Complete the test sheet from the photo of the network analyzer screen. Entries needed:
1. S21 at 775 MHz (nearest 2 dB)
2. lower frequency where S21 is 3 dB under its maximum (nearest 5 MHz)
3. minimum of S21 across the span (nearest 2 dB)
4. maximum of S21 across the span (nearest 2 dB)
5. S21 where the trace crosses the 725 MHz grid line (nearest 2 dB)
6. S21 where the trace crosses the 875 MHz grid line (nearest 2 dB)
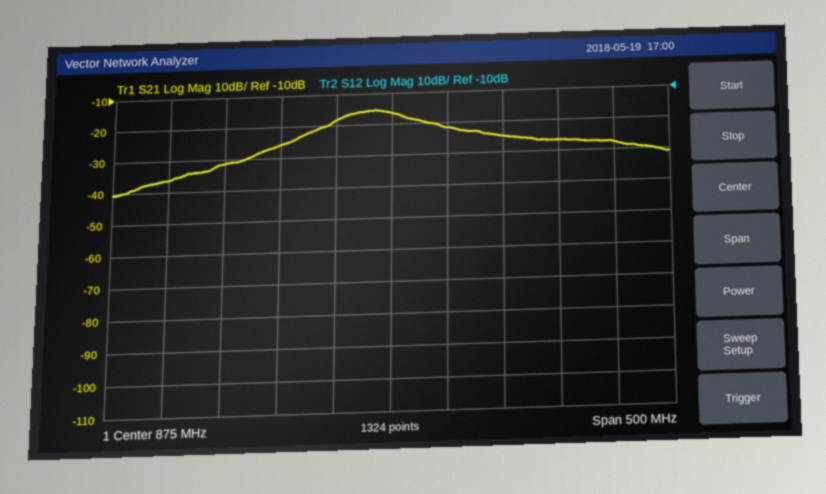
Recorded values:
-26 dB
825 MHz
-40 dB
-16 dB
-32 dB
-16 dB
